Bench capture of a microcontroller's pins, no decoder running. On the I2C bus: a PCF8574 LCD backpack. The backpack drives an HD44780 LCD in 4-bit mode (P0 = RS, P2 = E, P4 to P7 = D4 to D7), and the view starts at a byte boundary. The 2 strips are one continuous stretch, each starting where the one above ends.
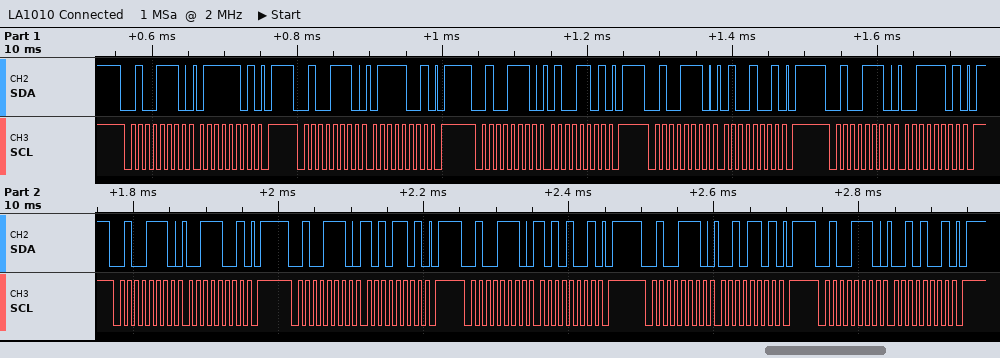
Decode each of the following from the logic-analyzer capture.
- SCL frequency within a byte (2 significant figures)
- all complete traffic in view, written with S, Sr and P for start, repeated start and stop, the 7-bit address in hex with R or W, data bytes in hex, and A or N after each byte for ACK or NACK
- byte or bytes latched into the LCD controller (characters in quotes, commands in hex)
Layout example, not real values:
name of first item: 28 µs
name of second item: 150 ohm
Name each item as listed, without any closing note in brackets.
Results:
SCL frequency within a byte: 100 kHz
all complete traffic in view, written with S, Sr and P for start, repeated start and stop, the 7-bit address in hex with R or W, data bytes in hex, and A or N after each byte for ACK or NACK: S 27W A 7D A P S 27W A 79 A P S 27W A 4D A P S 27W A 49 A P S 27W A 3D A P S 27W A 39 A P S 27W A AD A P S 27W A A9 A P S 27W A 2D A P S 27W A 29 A P
byte or bytes latched into the LCD controller: 't' ':'
